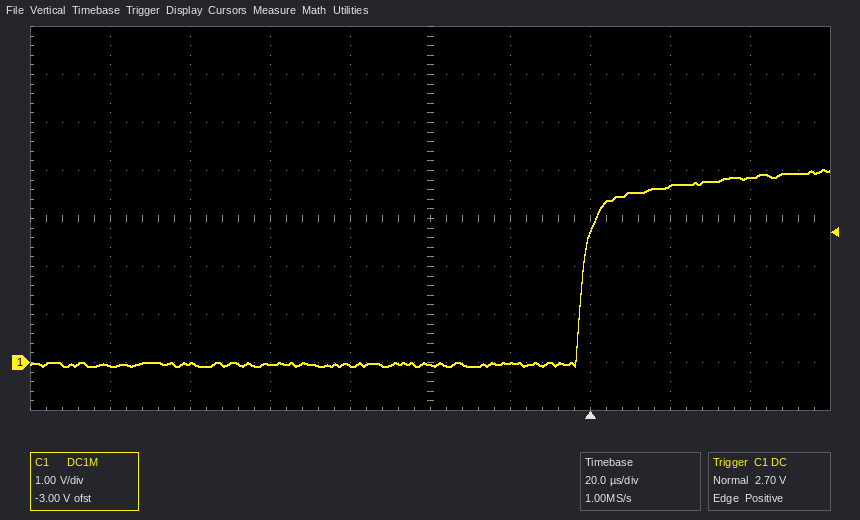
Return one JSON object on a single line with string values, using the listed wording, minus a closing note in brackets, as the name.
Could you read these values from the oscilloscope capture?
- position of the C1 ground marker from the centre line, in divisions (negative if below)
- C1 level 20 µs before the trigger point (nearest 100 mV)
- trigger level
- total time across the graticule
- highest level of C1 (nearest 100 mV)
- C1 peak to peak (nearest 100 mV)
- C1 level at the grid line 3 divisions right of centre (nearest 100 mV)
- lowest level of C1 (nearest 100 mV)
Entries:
{"position of the C1 ground marker from the centre line, in divisions": "-3.0 div", "C1 level 20 µs before the trigger point": "0.0 V", "trigger level": "2.70 V", "total time across the graticule": "200 µs", "highest level of C1": "4.0 V", "C1 peak to peak": "4.1 V", "C1 level at the grid line 3 divisions right of centre": "3.7 V", "lowest level of C1": "-100 mV"}
